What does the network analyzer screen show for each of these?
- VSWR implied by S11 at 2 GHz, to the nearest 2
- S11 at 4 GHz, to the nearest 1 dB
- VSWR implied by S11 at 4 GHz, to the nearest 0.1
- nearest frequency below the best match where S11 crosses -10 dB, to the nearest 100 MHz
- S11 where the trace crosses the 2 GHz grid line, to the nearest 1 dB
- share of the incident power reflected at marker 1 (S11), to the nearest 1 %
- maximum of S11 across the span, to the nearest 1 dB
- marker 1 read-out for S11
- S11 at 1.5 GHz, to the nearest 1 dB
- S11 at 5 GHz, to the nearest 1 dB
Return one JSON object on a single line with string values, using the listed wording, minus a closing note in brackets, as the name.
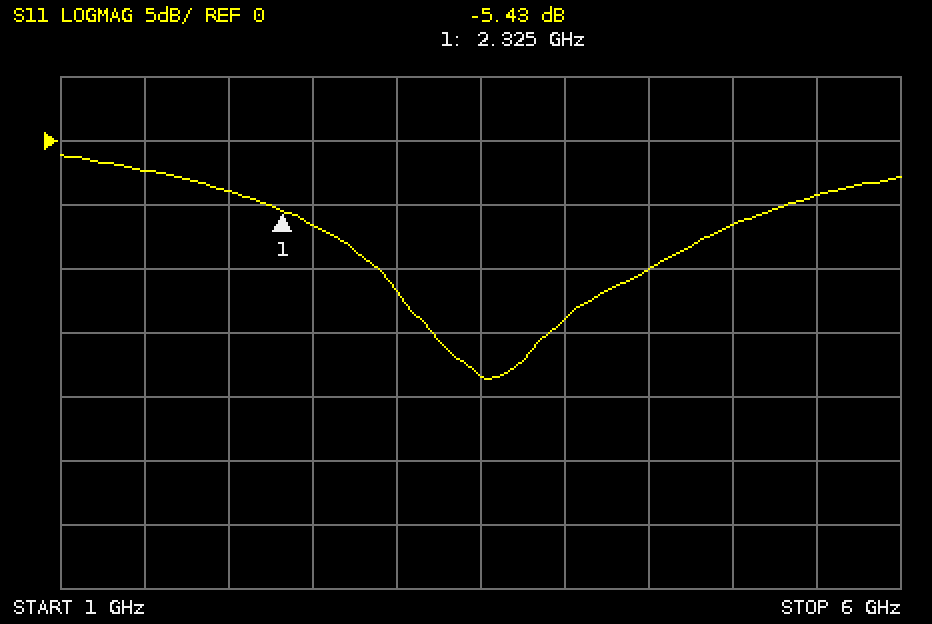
{"VSWR implied by S11 at 2 GHz, to the nearest 2": "4", "S11 at 4 GHz, to the nearest 1 dB": "-14 dB", "VSWR implied by S11 at 4 GHz, to the nearest 0.1": "1.5", "nearest frequency below the best match where S11 crosses -10 dB, to the nearest 100 MHz": "2.9 GHz", "S11 where the trace crosses the 2 GHz grid line, to the nearest 1 dB": "-4 dB", "share of the incident power reflected at marker 1 (S11), to the nearest 1 %": "29 %", "maximum of S11 across the span, to the nearest 1 dB": "-1 dB", "marker 1 read-out for S11": "-5.43 dB", "S11 at 1.5 GHz, to the nearest 1 dB": "-2 dB", "S11 at 5 GHz, to the nearest 1 dB": "-7 dB"}
